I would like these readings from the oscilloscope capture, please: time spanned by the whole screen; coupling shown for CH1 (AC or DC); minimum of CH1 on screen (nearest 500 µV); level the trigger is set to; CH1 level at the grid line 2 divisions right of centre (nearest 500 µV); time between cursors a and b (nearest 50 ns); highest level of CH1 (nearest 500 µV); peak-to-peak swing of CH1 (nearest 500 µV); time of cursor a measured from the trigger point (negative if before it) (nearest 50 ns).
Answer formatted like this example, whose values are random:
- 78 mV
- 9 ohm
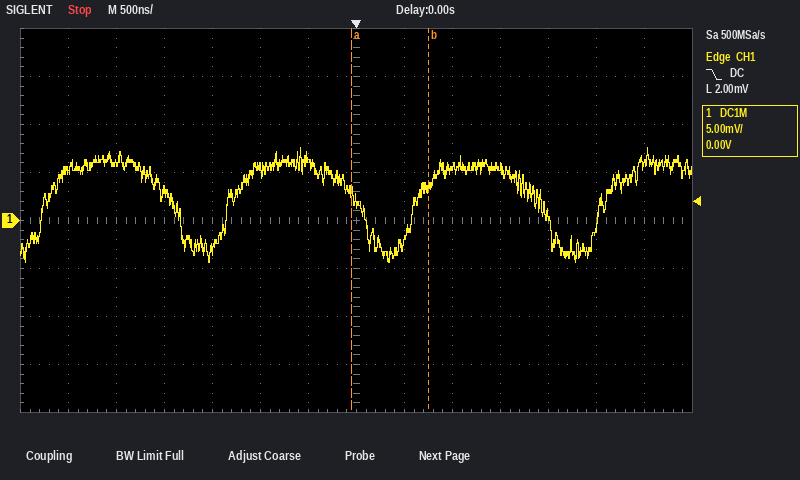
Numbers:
- 7 µs
- DC
- -4.5 mV
- 2.00 mV
- 5.5 mV
- 800 ns
- 7.5 mV
- 12.0 mV
- -50 ns
